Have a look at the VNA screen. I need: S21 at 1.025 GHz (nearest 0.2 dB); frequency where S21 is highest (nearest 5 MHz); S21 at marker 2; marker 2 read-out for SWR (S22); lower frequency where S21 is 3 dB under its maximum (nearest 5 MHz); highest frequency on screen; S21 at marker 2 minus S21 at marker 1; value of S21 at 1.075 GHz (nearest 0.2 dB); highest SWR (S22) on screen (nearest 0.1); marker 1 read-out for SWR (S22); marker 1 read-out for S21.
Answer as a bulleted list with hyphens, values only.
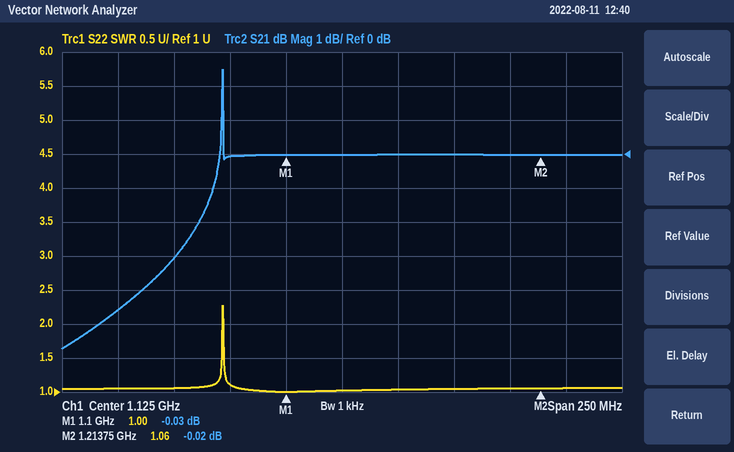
- -4.6 dB
- 1.070 GHz
- -0.02 dB
- 1.06
- 1.070 GHz
- 1.25 GHz
- 0.01 dB
- 0.0 dB
- 2.3
- 1.00
- -0.03 dB
